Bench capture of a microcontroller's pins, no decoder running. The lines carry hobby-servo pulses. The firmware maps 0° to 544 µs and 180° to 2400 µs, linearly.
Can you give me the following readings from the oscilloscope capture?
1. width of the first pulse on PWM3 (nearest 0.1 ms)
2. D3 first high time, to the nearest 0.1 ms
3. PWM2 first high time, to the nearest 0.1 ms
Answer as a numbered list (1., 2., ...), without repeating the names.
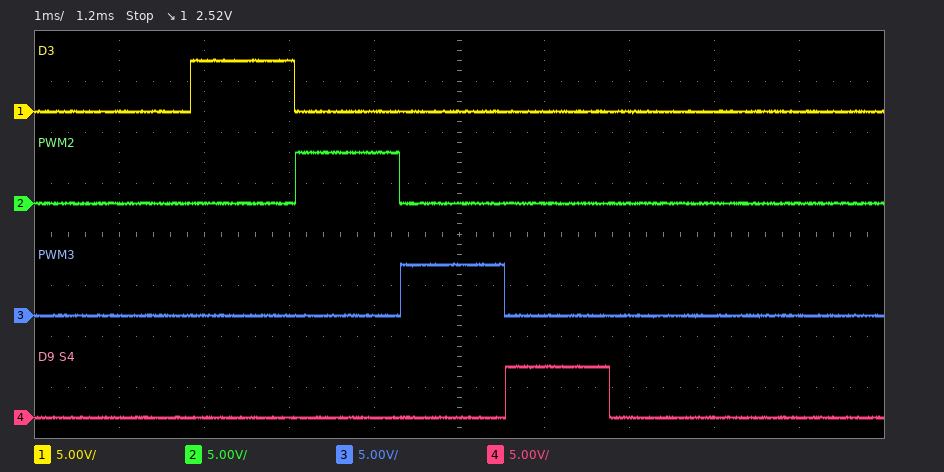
1. 1.2 ms
2. 1.2 ms
3. 1.2 ms
